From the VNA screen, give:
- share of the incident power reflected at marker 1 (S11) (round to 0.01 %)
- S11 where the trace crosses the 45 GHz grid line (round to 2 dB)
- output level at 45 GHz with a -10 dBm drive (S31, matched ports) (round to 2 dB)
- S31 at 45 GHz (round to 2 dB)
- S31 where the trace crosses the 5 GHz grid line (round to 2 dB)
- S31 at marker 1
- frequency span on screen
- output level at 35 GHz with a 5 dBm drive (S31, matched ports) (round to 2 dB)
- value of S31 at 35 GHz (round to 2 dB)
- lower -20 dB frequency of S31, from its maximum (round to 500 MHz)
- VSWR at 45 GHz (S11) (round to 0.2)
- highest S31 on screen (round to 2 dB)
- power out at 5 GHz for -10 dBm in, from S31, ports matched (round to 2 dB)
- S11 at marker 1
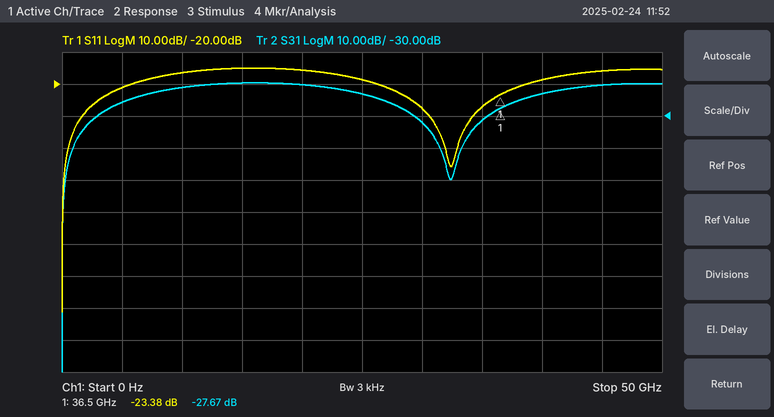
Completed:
0.46 %
-16 dB
-30 dBm
-20 dB
-26 dB
-27.67 dB
50 GHz
-26 dBm
-32 dB
1.0 GHz
1.4
-20 dB
-36 dBm
-23.38 dB
